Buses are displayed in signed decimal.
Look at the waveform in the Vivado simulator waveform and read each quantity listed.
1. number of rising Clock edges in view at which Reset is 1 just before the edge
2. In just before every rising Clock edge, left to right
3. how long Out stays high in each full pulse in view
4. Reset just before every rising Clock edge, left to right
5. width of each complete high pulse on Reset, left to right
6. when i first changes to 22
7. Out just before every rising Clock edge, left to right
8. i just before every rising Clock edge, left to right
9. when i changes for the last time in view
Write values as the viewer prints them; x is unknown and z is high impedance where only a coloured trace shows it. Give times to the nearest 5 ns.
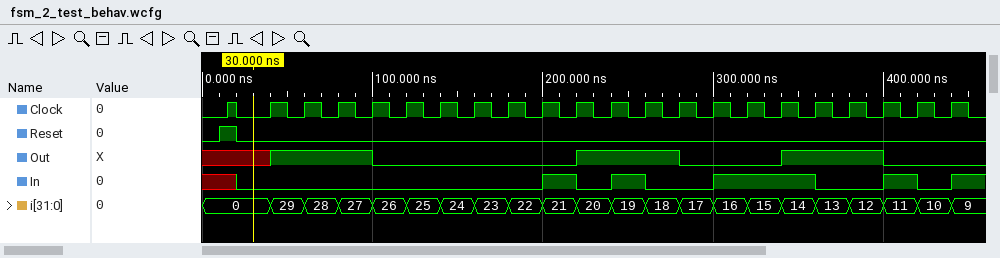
1
x 0 0 0 0 0 0 0 0 0 1 0 1 0 0 1 1 1 0 0 1 0
60 ns, 60 ns
1 0 0 0 0 0 0 0 0 0 0 0 0 0 0 0 0 0 0 0 0 0
10 ns
180 ns
x x 1 1 1 0 0 0 0 0 0 1 1 1 0 0 0 1 1 1 0 0
0, 0, 29, 28, 27, 26, 25, 24, 23, 22, 21, 20, 19, 18, 17, 16, 15, 14, 13, 12, 11, 10
440 ns
